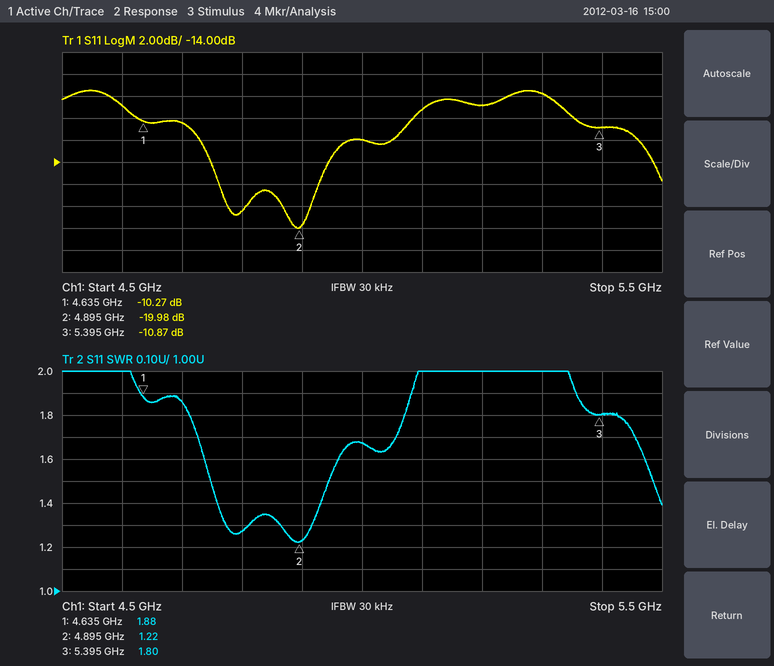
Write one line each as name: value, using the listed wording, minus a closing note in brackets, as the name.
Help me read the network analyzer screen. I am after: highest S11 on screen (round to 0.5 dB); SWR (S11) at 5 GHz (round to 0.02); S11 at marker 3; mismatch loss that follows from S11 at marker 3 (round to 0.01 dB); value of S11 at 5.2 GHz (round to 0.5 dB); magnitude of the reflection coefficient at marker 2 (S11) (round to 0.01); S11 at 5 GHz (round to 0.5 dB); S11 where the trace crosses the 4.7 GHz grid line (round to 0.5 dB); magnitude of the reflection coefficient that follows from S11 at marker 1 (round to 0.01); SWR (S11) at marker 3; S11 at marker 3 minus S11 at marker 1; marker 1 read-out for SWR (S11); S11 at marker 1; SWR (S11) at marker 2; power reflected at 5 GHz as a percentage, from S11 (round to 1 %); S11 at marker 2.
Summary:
highest S11 on screen: -7.5 dB
SWR (S11) at 5 GHz: 1.68
S11 at marker 3: -10.87 dB
mismatch loss that follows from S11 at marker 3: 0.37 dB
value of S11 at 5.2 GHz: -9.0 dB
magnitude of the reflection coefficient at marker 2 (S11): 0.10
S11 at 5 GHz: -12.0 dB
S11 where the trace crosses the 4.7 GHz grid line: -10.5 dB
magnitude of the reflection coefficient that follows from S11 at marker 1: 0.31
SWR (S11) at marker 3: 1.80
S11 at marker 3 minus S11 at marker 1: -0.60 dB
marker 1 read-out for SWR: 1.88
S11 at marker 1: -10.27 dB
SWR (S11) at marker 2: 1.22
power reflected at 5 GHz as a percentage, from S11: 6 %
S11 at marker 2: -19.98 dB
